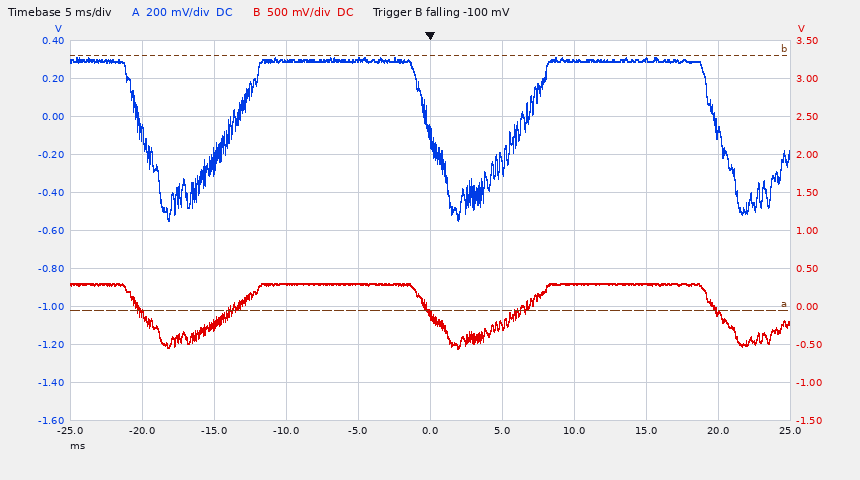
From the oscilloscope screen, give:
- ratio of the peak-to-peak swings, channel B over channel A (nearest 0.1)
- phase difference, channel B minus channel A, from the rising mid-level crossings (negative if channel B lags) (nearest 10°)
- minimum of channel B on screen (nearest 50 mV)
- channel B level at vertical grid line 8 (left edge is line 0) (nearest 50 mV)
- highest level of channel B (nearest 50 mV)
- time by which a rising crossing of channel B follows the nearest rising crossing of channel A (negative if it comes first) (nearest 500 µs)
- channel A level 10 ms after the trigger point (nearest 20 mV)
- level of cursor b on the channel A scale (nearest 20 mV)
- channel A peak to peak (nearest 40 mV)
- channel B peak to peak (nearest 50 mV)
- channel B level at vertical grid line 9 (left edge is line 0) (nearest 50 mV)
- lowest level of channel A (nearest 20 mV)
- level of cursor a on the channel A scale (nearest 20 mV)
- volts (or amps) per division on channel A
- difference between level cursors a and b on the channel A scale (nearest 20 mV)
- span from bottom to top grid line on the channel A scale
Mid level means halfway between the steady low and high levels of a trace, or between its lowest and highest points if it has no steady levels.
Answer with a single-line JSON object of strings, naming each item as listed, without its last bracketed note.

{"ratio of the peak-to-peak swings, channel B over channel A": "1.0", "phase difference, channel B minus channel A, from the rising mid-level crossings (negative if channel B lags)": "0°", "minimum of channel B on screen": "-550 mV", "channel B level at vertical grid line 8 (left edge is line 0)": "300 mV", "highest level of channel B": "300 mV", "time by which a rising crossing of channel B follows the nearest rising crossing of channel A (negative if it comes first)": "0.0 ms", "channel A level 10 ms after the trigger point": "300 mV", "level of cursor b on the channel A scale": "320 mV", "channel A peak to peak": "840 mV", "channel B peak to peak": "850 mV", "channel B level at vertical grid line 9 (left edge is line 0)": "-50 mV", "lowest level of channel A": "-540 mV", "level of cursor a on the channel A scale": "-1.02 V", "volts (or amps) per division on channel A": "200 mV", "difference between level cursors a and b on the channel A scale": "1.34 V", "span from bottom to top grid line on the channel A scale": "2 V"}
